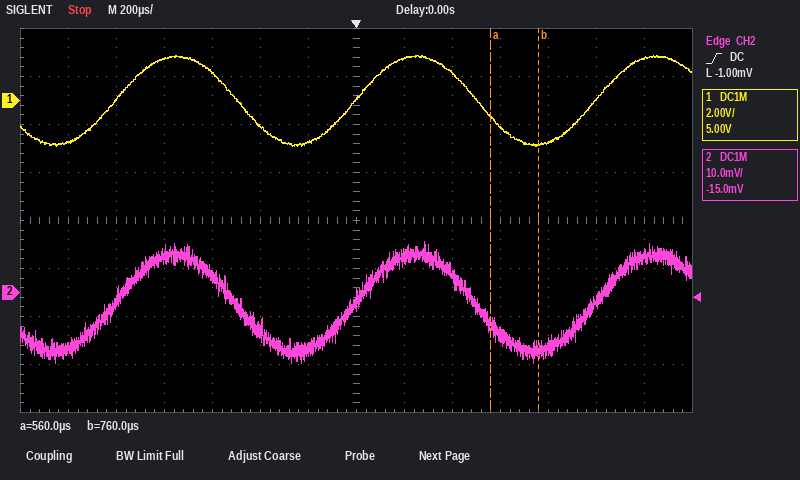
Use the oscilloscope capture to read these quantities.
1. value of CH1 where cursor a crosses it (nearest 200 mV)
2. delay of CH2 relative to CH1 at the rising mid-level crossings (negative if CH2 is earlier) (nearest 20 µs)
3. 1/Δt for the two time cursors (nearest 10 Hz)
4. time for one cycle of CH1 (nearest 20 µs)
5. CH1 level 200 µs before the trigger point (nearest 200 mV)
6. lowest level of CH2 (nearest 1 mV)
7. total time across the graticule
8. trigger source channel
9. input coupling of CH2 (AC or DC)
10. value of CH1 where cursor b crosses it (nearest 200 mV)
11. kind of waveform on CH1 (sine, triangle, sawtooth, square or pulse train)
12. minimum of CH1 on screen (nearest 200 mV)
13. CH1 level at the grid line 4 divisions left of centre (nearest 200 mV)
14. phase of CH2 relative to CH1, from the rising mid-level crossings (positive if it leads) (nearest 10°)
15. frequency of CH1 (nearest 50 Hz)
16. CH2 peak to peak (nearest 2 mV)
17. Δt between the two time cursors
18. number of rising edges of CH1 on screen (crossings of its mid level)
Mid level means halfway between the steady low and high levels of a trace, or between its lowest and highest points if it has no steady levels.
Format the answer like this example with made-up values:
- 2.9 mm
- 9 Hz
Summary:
- -600 mV
- 0 µs
- 5.00 kHz
- 1.00 ms
- -1.8 V
- -15 mV
- 2.8 ms
- CH2
- DC
- -1.8 V
- sine
- -2.0 V
- 1.8 V
- 0°
- 1.00 kHz
- 26 mV
- 200 µs
- 3
